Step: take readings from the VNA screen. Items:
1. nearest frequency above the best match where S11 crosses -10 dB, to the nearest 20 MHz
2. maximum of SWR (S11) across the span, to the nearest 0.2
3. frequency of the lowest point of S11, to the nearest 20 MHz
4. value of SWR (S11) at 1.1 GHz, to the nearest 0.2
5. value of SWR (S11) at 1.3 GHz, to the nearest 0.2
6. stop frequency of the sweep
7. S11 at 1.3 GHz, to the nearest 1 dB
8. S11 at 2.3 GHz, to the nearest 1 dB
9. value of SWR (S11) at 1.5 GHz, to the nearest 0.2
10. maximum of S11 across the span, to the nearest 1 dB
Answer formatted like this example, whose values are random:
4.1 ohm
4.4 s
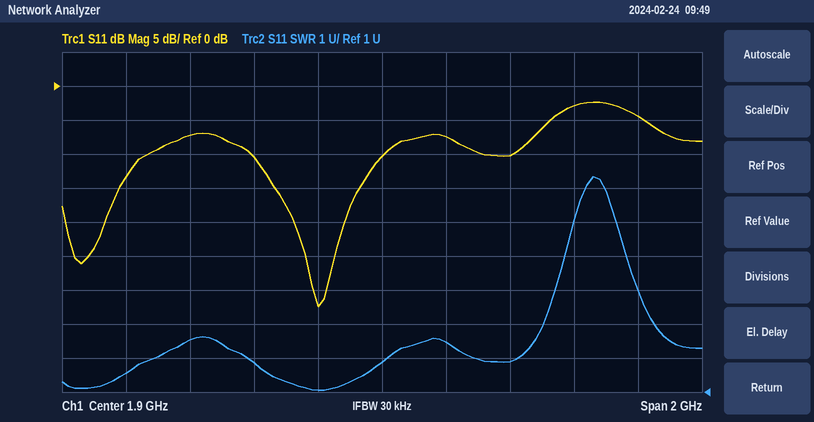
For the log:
1.90 GHz
7.4
1.70 GHz
1.6
2.6
2.9 GHz
-7 dB
-10 dB
1.8
-2 dB
